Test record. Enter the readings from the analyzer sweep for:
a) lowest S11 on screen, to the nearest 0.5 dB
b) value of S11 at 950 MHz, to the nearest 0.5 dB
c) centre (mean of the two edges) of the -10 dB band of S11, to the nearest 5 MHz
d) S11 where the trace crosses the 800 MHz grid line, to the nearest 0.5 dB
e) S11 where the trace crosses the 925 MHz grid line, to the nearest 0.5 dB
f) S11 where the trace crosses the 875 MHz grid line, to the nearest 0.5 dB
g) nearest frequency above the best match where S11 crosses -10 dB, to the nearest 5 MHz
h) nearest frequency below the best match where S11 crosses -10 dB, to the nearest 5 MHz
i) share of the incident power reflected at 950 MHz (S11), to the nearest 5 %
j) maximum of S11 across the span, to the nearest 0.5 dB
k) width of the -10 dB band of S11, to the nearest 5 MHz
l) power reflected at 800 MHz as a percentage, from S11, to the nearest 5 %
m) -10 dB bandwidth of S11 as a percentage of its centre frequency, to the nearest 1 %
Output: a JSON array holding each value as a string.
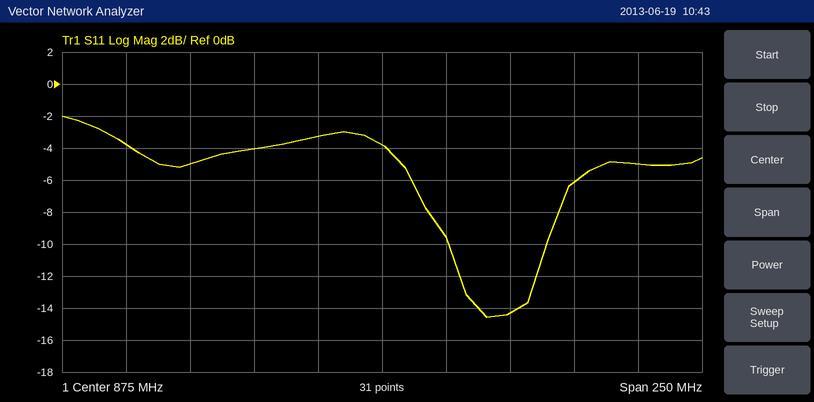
["-14.5 dB", "-6.0 dB", "920 MHz", "-5.0 dB", "-14.5 dB", "-4.0 dB", "940 MHz", "900 MHz", "25 %", "-2.0 dB", "40 MHz", "30 %", "4 %"]
